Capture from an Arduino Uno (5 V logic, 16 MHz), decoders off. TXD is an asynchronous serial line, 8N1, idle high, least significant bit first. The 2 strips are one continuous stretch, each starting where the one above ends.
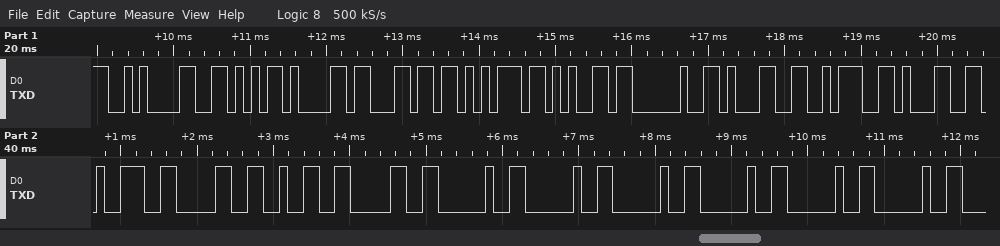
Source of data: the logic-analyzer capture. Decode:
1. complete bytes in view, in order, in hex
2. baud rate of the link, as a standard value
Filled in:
0x0A 0x56 0x61 0x6C 0x75 0x65 0x20 0x31 0x3A 0x31 0x39 0x30 0x32 0x30 0x20 0x20 0x20 0x20 0x20 0x20
9600 baud
